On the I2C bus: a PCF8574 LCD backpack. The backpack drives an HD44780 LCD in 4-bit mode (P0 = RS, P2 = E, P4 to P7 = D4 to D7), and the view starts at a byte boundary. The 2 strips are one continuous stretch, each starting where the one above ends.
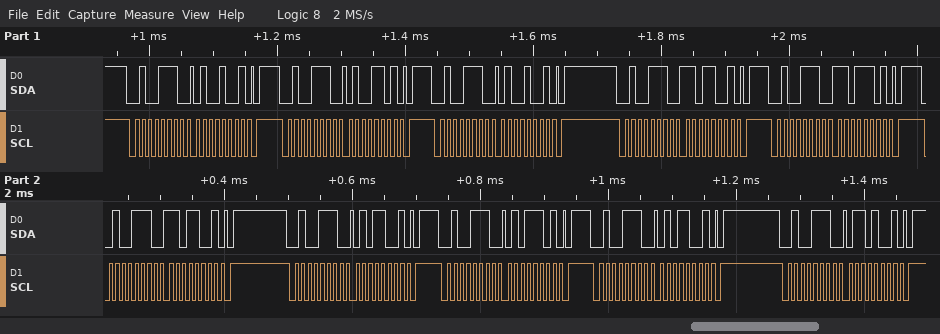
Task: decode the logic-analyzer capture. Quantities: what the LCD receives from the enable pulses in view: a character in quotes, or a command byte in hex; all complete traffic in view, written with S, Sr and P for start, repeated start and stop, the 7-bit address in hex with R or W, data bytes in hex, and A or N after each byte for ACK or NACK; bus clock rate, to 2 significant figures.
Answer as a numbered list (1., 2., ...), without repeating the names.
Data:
1. 'M'
2. S 27W A 49 A P S 27W A 4D A P S 27W A 49 A P S 27W A D9 A P S 27W A DD A P S 27W A D9 A P S 27W A 59 A P S 27W A 5D A P S 27W A 59 A P S 27W A 69 A P
3. 100 kHz
